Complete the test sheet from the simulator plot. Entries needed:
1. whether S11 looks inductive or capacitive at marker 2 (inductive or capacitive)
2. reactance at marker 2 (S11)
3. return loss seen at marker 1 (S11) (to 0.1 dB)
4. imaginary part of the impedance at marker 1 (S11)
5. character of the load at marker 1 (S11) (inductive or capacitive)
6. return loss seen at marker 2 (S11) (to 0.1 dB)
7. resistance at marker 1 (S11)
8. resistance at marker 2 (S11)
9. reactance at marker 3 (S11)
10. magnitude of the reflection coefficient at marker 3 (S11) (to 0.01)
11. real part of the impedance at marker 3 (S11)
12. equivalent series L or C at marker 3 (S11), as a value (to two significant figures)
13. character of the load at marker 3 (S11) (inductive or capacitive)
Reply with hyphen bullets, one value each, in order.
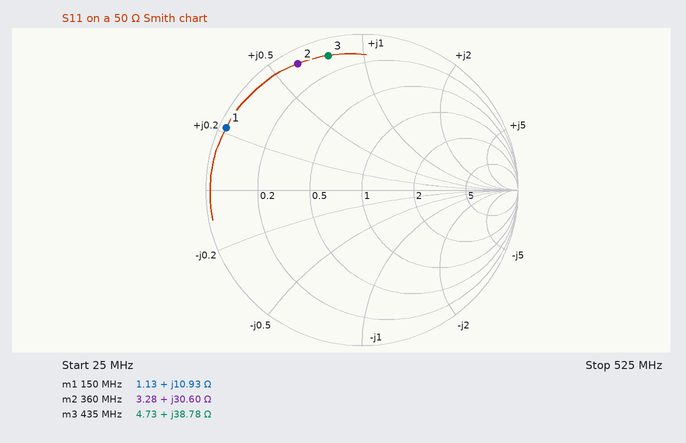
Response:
- inductive
- +30.60 Ω
- 0.4 dB
- +10.93 Ω
- inductive
- 0.8 dB
- 1.13 Ω
- 3.28 Ω
- +38.78 Ω
- 0.89
- 4.73 Ω
- 14 nH
- inductive
